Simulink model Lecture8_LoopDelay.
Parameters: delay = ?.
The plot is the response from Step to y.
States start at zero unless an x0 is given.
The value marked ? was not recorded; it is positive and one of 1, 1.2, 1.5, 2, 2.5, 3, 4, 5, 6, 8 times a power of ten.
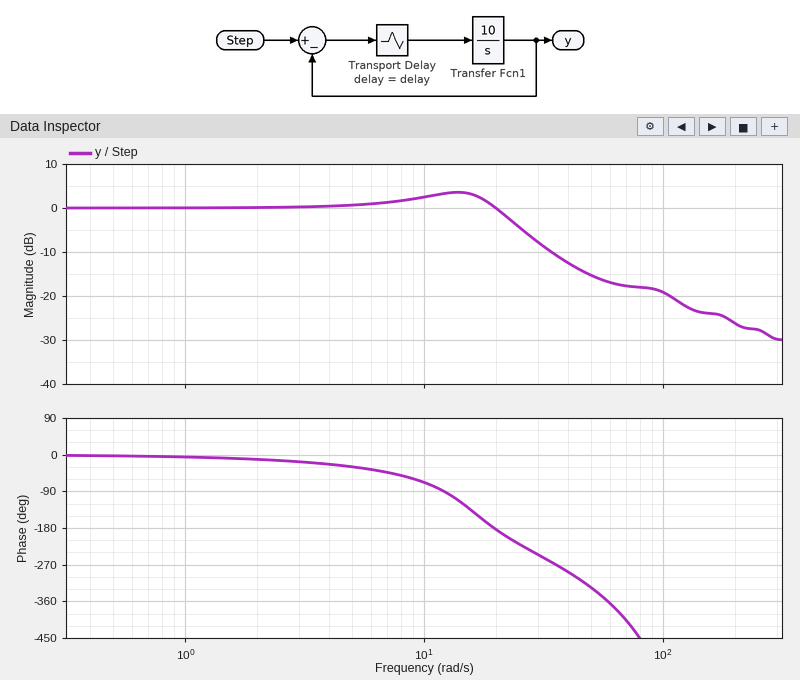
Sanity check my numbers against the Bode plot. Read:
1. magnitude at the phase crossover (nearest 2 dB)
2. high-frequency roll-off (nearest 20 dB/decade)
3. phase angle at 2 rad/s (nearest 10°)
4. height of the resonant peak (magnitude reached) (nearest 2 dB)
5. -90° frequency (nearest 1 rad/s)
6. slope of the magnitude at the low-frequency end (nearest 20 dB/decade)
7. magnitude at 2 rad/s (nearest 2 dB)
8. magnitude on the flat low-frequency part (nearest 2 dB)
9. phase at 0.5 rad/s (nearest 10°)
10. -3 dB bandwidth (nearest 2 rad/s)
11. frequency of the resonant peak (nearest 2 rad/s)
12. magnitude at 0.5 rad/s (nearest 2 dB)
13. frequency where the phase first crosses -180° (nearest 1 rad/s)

0 dB
-20 dB/decade
-10°
4 dB
12 rad/s
0 dB/decade
0 dB
0 dB
0°
24 rad/s
14 rad/s
0 dB
20 rad/s
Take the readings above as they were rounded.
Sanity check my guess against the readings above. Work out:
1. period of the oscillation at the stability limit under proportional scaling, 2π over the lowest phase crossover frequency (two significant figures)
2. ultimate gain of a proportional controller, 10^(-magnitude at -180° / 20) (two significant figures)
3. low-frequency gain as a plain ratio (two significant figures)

0.31 s
1.0
1.0
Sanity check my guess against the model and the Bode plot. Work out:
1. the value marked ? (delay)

0.08
